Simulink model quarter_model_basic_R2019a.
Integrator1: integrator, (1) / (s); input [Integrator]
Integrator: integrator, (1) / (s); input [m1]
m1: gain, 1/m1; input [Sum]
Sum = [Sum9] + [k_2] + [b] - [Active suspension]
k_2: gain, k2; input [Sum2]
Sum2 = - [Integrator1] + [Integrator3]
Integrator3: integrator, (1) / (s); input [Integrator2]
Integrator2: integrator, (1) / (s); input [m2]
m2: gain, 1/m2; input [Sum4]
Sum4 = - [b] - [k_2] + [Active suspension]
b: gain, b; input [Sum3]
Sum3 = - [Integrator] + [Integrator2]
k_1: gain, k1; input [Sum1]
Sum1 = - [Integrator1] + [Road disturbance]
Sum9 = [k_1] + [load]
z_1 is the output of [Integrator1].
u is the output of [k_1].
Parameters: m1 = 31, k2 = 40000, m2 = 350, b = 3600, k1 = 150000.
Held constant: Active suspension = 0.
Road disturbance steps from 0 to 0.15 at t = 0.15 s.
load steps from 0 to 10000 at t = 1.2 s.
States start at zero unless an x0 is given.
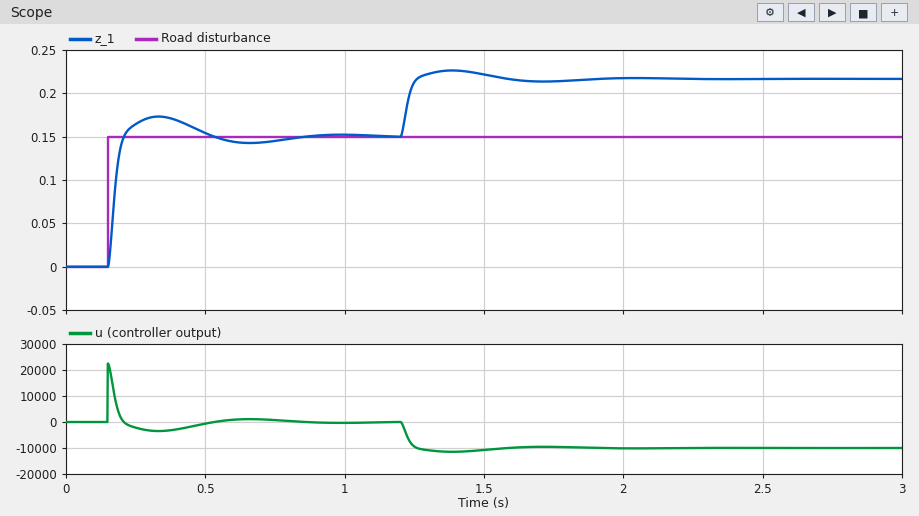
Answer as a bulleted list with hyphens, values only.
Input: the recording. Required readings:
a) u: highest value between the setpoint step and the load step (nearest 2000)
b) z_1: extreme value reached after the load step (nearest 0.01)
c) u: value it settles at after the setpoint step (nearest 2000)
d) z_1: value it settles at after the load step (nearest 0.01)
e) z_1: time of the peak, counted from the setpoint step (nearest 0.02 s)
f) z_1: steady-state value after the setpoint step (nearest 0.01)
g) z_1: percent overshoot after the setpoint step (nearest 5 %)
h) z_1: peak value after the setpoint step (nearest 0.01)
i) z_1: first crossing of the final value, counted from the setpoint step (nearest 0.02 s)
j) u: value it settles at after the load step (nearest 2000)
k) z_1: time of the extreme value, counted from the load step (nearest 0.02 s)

- 22000
- 0.23
- 0
- 0.22
- 0.18 s
- 0.15
- 15 %
- 0.17
- 0.06 s
- -10000
- 0.18 s
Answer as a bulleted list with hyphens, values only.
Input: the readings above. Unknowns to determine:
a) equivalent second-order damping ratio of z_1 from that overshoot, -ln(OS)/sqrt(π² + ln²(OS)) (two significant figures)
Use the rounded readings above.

- 0.52
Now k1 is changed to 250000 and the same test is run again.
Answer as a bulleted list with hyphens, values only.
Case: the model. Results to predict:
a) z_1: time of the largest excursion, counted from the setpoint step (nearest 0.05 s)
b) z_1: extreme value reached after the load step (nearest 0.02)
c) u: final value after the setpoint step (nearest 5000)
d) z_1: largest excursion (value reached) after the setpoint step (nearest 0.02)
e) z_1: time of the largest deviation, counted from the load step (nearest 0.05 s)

- 0.15 s
- 0.20
- 0
- 0.16
- 0.15 s
